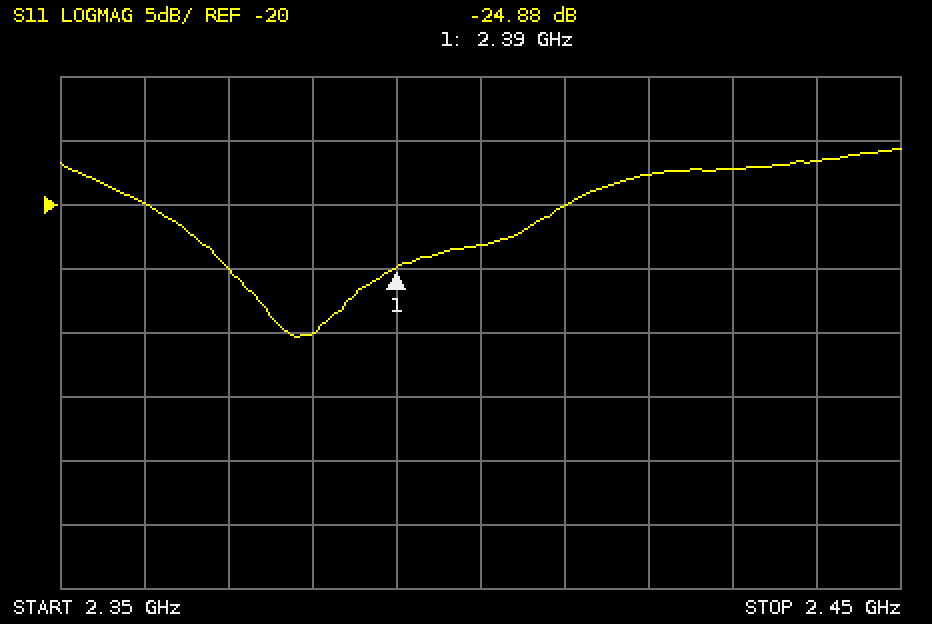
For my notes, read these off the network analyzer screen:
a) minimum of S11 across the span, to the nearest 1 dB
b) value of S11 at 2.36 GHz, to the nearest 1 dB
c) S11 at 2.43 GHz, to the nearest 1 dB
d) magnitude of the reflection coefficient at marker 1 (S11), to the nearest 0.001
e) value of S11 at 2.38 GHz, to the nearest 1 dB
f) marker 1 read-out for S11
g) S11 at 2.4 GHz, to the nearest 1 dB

-30 dB
-20 dB
-17 dB
0.057
-30 dB
-24.88 dB
-23 dB
